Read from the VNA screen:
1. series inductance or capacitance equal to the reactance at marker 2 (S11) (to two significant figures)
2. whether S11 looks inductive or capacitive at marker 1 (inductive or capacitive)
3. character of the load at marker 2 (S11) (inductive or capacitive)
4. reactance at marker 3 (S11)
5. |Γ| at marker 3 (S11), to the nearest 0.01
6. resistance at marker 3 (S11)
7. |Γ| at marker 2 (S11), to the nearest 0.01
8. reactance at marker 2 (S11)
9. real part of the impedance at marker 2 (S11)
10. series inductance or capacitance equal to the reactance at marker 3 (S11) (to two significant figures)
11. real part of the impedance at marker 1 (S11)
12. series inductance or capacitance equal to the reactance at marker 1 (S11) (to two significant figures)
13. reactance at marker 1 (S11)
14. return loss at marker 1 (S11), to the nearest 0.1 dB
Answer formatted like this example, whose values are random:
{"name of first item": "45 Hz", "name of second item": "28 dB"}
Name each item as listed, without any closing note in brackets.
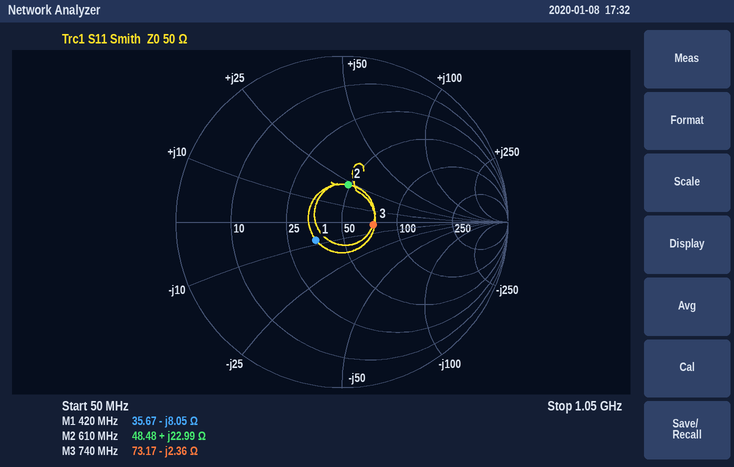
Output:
{"series inductance or capacitance equal to the reactance at marker 2 (S11)": "6.0 nH", "whether S11 looks inductive or capacitive at marker 1": "capacitive", "character of the load at marker 2 (S11)": "inductive", "reactance at marker 3": "-2.36 Ω", "|Γ| at marker 3 (S11), to the nearest 0.01": "0.19", "resistance at marker 3": "73.17 Ω", "|Γ| at marker 2 (S11), to the nearest 0.01": "0.23", "reactance at marker 2": "+22.99 Ω", "real part of the impedance at marker 2": "48.48 Ω", "series inductance or capacitance equal to the reactance at marker 3 (S11)": "91 pF", "real part of the impedance at marker 1": "35.67 Ω", "series inductance or capacitance equal to the reactance at marker 1 (S11)": "47 pF", "reactance at marker 1": "-8.05 Ω", "return loss at marker 1 (S11), to the nearest 0.1 dB": "14.4 dB"}
